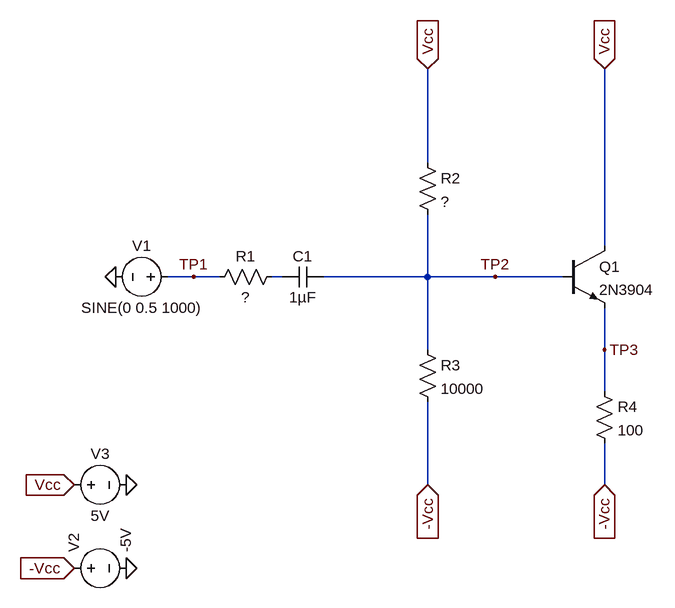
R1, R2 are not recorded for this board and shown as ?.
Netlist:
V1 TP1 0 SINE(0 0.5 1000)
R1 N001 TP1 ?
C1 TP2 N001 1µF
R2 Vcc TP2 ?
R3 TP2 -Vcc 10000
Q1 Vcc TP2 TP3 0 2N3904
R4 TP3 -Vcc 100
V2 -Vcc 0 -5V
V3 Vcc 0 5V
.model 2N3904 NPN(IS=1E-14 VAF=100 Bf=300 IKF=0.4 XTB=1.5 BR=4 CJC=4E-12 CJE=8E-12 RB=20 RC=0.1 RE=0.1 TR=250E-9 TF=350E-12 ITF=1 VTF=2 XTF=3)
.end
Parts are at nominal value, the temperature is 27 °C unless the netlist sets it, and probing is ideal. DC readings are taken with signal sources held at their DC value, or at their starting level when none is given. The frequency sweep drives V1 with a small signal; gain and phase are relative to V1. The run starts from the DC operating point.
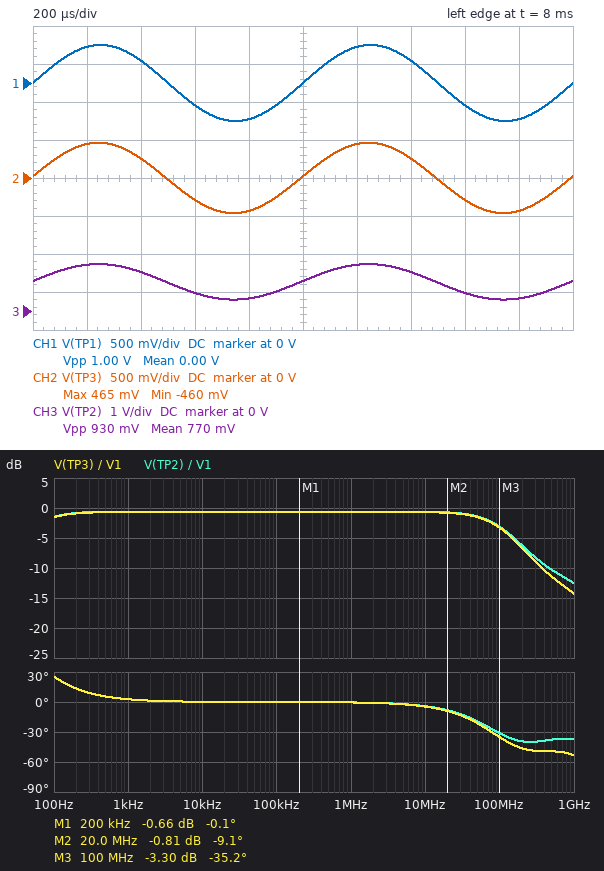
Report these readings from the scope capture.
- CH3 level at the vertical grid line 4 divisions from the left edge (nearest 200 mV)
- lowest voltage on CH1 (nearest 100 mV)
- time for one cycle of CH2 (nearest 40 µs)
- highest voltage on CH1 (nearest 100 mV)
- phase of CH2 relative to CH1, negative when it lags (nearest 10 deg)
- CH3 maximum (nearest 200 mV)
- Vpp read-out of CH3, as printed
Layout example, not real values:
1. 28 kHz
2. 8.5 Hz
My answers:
1. 400 mV
2. -500 mV
3. 1.00 ms
4. 500 mV
5. 0 deg
6. 1.2 V
7. 930 mV
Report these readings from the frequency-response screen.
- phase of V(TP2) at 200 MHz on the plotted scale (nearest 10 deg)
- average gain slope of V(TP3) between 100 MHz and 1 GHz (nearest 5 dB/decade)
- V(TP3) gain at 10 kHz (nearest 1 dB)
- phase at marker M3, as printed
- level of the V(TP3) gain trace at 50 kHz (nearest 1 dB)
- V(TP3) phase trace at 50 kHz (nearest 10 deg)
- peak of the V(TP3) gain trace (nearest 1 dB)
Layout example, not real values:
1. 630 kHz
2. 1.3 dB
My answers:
1. -40 deg
2. -10 dB/decade
3. -1 dB
4. -35.2 deg
5. -1 dB
6. 0 deg
7. -1 dB
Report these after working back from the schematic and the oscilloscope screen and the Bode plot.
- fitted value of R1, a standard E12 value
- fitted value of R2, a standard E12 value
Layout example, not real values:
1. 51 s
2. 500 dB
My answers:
1. 220 Ω
2. 5.6 kΩ
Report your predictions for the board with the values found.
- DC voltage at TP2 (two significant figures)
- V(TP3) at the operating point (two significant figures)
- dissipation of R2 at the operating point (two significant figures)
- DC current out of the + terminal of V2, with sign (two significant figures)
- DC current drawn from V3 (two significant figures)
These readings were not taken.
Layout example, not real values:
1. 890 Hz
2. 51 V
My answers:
1. 770 mV
2. 2.9 mV
3. 3.2 mW
4. -51 mA
5. 51 mA
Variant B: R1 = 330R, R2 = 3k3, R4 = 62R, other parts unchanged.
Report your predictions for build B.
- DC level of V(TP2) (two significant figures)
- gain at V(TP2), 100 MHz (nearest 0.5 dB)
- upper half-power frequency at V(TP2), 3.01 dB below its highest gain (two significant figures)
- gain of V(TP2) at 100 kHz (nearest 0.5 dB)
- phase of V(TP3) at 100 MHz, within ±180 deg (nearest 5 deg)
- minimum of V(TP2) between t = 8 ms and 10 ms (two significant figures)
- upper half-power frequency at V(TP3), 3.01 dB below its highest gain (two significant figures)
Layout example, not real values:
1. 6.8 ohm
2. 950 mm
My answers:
1. 1.6 V
2. -7.0 dB
3. 60 MHz
4. -1.5 dB
5. -50 deg
6. 1.2 V
7. 59 MHz
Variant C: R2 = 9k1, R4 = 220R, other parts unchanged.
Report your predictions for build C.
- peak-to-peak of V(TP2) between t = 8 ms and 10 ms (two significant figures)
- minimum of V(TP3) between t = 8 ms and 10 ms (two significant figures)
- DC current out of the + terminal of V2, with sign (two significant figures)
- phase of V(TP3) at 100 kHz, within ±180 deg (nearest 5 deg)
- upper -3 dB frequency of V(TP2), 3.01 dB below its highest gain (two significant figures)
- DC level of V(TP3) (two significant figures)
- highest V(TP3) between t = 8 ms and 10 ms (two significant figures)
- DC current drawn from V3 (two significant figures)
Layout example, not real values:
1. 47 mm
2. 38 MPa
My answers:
1. 950 mV
2. -1.3 V
3. -20 mA
4. 0 deg
5. 170 MHz
6. -800 mV
7. -330 mV
8. 20 mA
